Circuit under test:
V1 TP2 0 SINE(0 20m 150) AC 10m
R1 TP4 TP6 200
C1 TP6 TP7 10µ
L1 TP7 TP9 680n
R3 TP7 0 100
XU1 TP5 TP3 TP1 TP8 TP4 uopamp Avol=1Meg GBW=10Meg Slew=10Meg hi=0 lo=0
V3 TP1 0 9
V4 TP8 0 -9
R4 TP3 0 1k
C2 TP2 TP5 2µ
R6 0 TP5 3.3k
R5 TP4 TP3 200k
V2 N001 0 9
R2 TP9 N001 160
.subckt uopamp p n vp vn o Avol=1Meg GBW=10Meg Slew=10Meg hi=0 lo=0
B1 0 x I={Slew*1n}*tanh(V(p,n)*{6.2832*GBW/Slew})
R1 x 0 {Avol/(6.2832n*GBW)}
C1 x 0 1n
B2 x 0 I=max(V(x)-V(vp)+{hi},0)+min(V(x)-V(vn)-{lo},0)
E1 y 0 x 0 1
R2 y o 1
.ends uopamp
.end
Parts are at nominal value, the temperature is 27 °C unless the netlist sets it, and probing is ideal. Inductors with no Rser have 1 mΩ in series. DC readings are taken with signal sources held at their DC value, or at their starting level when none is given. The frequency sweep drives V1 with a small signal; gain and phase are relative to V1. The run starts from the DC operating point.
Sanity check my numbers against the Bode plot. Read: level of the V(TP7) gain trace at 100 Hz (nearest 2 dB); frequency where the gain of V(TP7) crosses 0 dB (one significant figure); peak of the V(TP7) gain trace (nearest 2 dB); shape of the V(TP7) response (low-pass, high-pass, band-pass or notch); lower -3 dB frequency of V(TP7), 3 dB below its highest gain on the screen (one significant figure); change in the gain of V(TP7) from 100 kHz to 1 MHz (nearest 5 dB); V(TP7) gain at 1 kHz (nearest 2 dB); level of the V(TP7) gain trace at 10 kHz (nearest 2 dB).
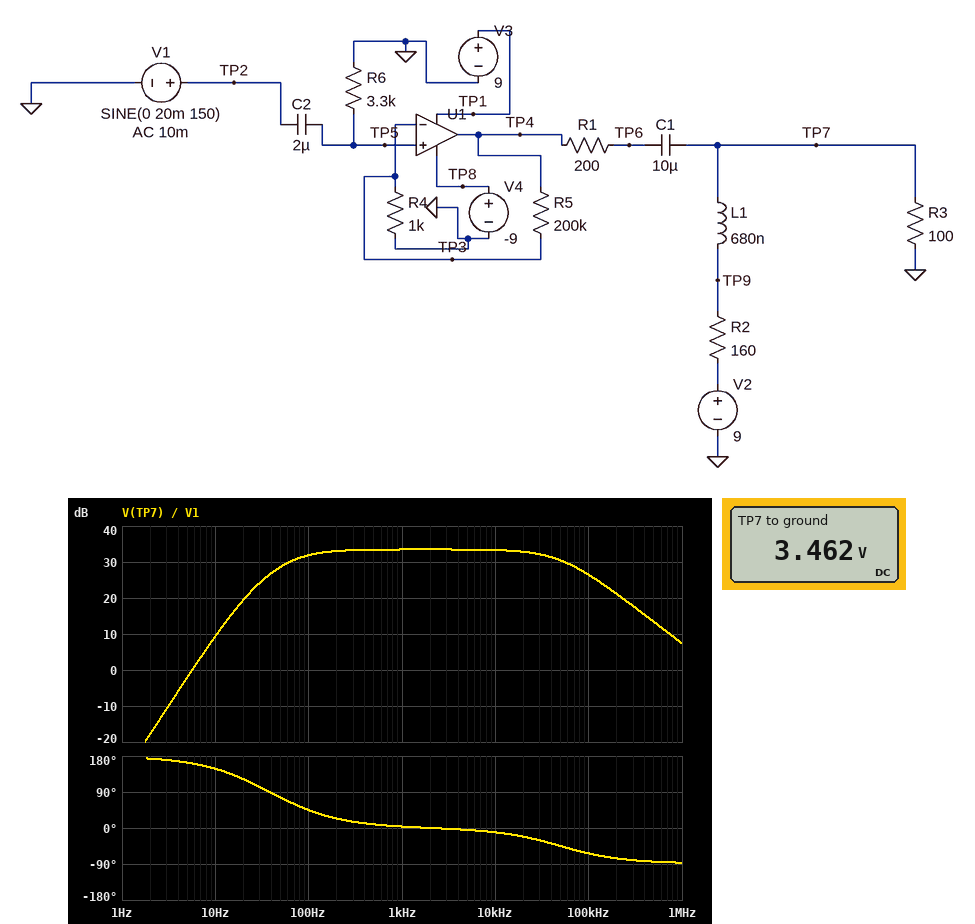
32 dB
6 Hz
34 dB
band-pass
70 Hz
-20 dB
34 dB
34 dB
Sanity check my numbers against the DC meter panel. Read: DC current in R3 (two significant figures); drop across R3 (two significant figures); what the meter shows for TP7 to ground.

35 mA
3.5 V
3.462 V
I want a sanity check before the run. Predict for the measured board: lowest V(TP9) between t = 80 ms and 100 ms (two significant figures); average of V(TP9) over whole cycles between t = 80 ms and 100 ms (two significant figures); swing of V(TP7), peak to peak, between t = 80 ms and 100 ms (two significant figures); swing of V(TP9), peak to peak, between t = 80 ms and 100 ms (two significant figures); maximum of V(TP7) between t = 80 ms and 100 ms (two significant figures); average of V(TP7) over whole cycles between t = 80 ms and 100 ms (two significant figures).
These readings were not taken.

2.6 V
3.5 V
1.7 V
1.7 V
4.3 V
3.5 V
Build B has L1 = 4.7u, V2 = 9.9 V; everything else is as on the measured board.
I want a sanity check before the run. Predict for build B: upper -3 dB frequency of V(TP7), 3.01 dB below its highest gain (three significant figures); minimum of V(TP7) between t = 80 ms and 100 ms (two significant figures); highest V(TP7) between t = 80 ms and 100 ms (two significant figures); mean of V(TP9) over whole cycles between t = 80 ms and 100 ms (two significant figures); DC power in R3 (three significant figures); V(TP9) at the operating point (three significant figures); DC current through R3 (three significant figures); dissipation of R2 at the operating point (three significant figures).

49.7 kHz
2.9 V
4.7 V
3.8 V
145 mW
3.81 V
38.1 mA
232 mW
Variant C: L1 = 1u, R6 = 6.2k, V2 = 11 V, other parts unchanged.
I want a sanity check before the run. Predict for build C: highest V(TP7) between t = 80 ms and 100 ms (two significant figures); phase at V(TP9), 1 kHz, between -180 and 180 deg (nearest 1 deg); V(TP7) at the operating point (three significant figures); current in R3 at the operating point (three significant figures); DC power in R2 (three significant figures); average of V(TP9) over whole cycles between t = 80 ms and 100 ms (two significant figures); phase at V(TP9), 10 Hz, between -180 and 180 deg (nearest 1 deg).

5.1 V
3 deg
4.23 V
42.3 mA
286 mW
4.2 V
133 deg
